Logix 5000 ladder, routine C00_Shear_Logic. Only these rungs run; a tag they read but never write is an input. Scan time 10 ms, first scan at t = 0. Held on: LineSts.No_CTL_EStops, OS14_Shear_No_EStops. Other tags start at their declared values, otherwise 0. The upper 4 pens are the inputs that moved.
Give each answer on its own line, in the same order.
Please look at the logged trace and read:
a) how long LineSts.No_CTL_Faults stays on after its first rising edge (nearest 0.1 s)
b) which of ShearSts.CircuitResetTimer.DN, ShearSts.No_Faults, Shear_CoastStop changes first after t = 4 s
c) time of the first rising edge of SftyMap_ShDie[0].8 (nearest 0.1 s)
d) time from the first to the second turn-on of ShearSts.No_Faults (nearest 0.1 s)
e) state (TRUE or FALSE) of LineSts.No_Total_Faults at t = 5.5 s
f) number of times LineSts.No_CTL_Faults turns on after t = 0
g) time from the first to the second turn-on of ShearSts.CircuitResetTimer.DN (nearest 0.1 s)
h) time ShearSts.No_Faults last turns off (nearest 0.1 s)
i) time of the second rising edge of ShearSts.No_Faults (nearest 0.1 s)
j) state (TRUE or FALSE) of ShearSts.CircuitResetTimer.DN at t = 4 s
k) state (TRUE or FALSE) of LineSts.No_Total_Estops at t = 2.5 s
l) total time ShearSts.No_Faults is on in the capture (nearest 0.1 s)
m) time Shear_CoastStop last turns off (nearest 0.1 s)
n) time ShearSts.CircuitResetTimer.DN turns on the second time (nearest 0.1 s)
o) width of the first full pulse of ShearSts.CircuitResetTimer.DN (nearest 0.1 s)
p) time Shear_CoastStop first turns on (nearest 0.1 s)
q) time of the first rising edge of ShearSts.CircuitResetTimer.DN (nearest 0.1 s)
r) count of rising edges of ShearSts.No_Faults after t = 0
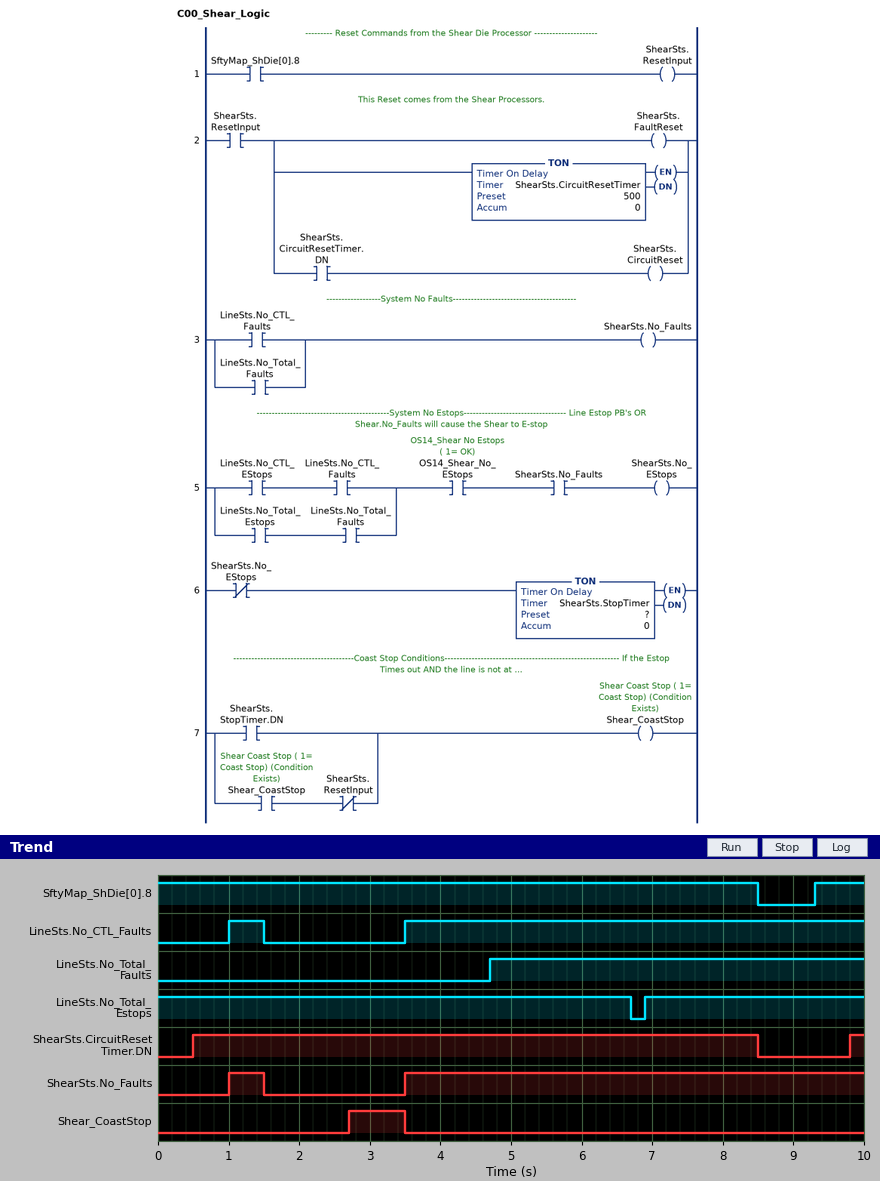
0.5 s
ShearSts.CircuitResetTimer.DN
9.3 s
2.5 s
TRUE
2
9.3 s
1.5 s
3.5 s
TRUE
TRUE
7.0 s
3.5 s
9.8 s
8.0 s
2.7 s
0.5 s
2
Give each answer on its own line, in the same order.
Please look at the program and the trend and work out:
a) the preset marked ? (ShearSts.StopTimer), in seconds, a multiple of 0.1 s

1.2 s
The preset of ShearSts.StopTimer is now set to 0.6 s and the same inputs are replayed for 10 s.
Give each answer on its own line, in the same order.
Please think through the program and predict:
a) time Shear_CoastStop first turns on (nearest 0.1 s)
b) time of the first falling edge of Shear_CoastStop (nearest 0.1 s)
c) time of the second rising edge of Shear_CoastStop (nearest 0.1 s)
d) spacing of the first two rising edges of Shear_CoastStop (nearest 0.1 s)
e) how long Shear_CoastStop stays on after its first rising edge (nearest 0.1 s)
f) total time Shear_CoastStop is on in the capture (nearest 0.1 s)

0.6 s
1.0 s
2.1 s
1.5 s
0.4 s
1.8 s
